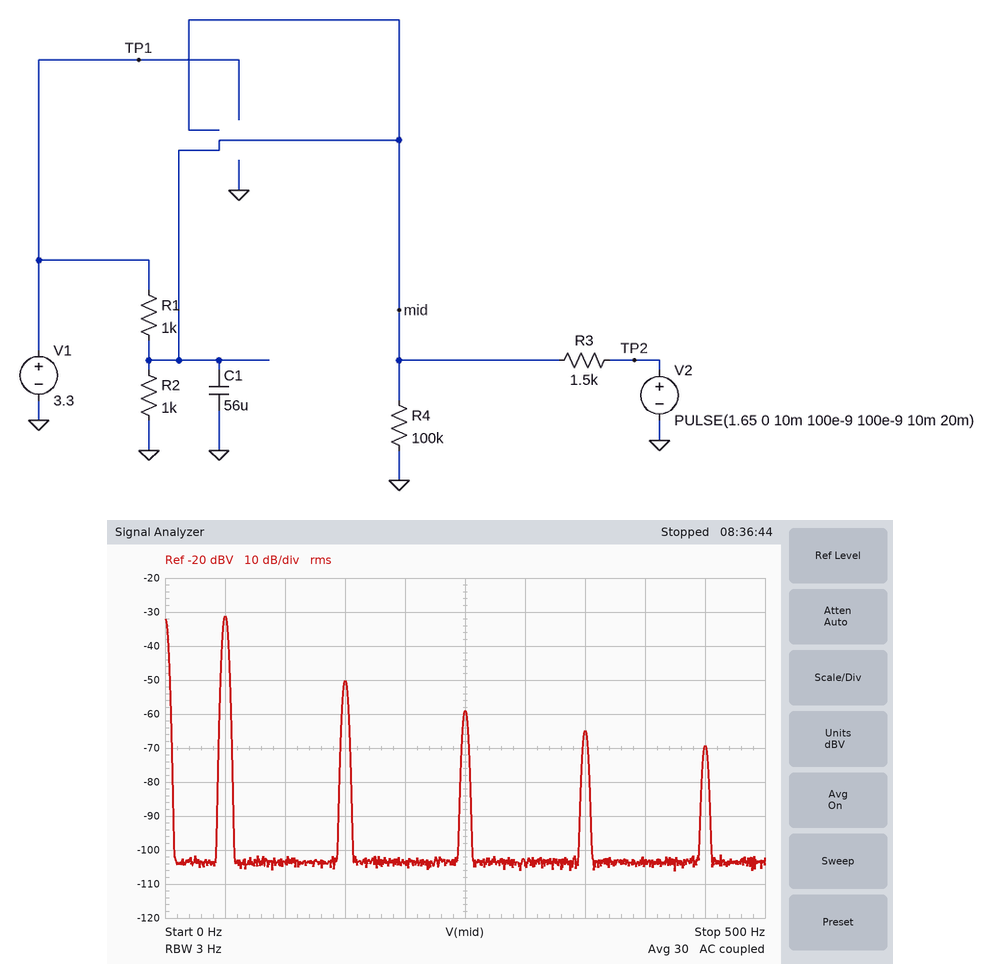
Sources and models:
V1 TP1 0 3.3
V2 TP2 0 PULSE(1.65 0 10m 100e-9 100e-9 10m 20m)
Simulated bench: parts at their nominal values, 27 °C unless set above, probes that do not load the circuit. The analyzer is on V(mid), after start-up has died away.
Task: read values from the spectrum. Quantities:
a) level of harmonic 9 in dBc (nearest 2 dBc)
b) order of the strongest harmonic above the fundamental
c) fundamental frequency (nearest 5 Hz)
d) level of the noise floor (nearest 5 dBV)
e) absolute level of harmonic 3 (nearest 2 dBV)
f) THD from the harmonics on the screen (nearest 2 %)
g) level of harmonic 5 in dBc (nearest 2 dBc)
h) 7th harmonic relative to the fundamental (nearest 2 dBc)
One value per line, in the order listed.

-38 dBc
3
50 Hz
-105 dBV
-50 dBV
12 %
-28 dBc
-34 dBc
